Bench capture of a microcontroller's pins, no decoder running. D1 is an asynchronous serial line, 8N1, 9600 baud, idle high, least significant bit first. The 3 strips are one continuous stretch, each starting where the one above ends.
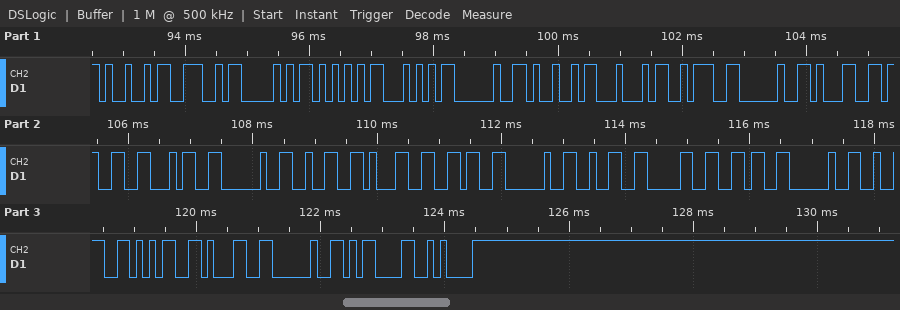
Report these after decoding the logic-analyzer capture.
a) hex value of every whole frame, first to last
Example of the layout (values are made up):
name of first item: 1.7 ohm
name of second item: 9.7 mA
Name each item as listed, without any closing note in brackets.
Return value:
hex value of every whole frame, first to last: 49 4E 50 55 54 20 49 44 3A 20 31 33 34 20 32 31 36 20 32 30 36 20 32 35 31 20 0D 0A
